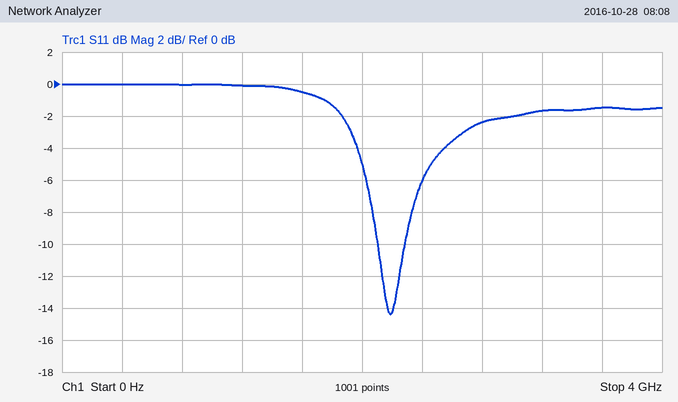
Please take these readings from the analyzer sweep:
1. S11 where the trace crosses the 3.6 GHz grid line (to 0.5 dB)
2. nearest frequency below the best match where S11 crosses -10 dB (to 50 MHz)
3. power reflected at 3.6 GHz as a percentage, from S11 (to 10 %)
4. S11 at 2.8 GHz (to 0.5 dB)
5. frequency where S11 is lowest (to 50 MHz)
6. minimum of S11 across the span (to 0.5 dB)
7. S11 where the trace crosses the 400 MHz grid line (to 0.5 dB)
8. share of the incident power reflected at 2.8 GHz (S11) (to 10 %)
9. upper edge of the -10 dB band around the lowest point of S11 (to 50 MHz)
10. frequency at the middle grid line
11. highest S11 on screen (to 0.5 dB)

-1.5 dB
2.10 GHz
70 %
-2.5 dB
2.20 GHz
-14.5 dB
0.0 dB
60 %
2.30 GHz
2 GHz
0.0 dB
